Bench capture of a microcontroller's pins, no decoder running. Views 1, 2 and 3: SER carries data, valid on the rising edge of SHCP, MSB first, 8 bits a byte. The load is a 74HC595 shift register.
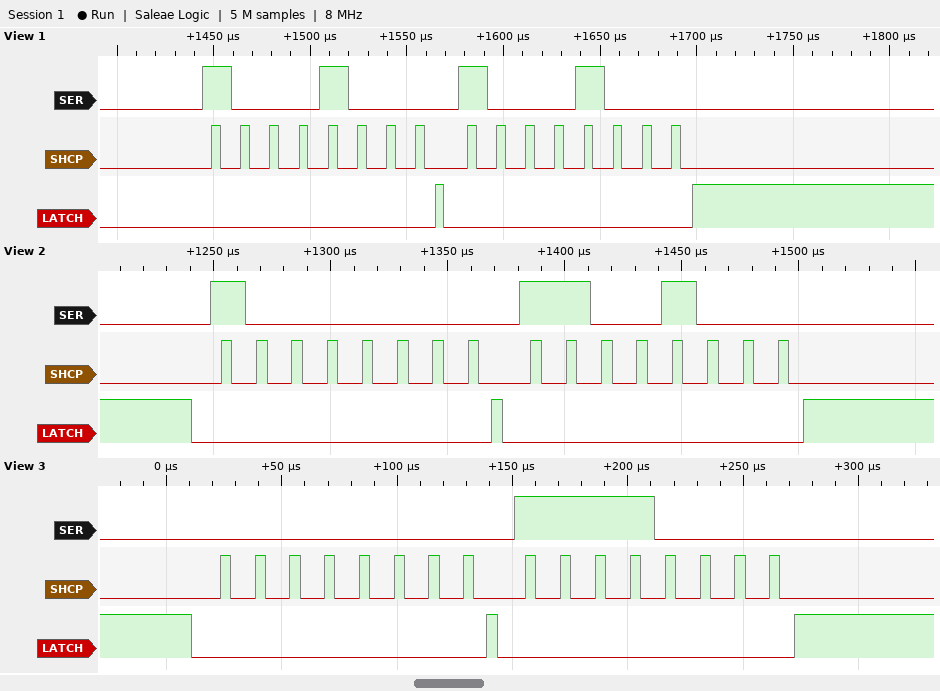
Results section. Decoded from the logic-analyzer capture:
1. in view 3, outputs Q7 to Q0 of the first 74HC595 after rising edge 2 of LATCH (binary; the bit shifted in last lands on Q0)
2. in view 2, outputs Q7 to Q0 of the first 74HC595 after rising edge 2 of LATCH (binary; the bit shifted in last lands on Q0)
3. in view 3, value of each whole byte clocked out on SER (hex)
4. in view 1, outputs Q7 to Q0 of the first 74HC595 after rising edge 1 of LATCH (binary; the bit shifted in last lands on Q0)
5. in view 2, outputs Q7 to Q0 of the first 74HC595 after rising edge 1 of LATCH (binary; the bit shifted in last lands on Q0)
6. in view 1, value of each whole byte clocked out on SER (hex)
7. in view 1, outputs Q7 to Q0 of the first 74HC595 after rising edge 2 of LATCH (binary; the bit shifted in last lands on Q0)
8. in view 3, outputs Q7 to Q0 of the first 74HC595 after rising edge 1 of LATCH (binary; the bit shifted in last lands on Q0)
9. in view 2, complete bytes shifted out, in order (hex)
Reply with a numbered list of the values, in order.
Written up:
1. 11110000
2. 11001000
3. 00 F0
4. 10001000
5. 10000000
6. 0x88 0x88
7. 10001000
8. 00000000
9. 80 C8
